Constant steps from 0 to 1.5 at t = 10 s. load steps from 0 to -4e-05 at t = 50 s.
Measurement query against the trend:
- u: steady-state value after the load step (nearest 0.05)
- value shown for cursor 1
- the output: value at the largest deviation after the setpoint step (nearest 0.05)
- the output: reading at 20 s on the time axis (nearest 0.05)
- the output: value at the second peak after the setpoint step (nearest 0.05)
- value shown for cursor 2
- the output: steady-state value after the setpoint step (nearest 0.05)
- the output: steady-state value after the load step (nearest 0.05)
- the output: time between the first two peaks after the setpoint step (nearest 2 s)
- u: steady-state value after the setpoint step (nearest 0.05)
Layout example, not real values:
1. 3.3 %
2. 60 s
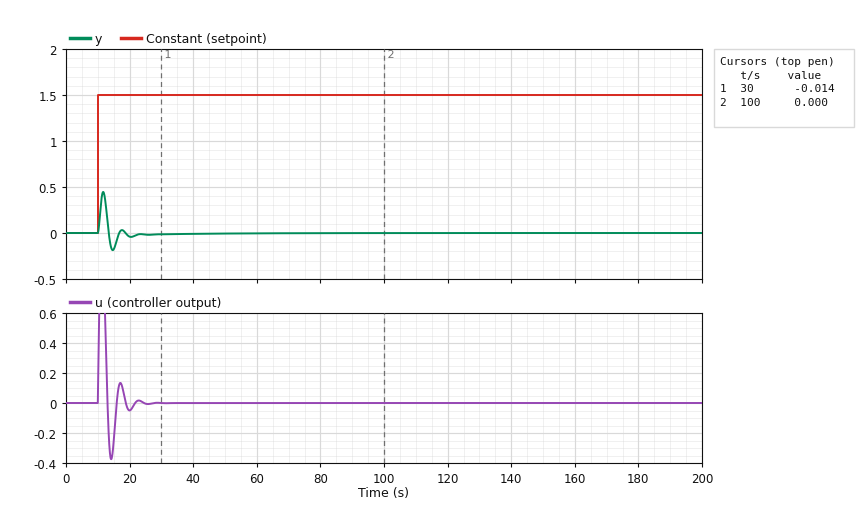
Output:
1. 0.00
2. -0.014
3. 0.45
4. -0.05
5. 0.05
6. 0.000
7. 0.00
8. 0.00
9. 6 s
10. 0.00
